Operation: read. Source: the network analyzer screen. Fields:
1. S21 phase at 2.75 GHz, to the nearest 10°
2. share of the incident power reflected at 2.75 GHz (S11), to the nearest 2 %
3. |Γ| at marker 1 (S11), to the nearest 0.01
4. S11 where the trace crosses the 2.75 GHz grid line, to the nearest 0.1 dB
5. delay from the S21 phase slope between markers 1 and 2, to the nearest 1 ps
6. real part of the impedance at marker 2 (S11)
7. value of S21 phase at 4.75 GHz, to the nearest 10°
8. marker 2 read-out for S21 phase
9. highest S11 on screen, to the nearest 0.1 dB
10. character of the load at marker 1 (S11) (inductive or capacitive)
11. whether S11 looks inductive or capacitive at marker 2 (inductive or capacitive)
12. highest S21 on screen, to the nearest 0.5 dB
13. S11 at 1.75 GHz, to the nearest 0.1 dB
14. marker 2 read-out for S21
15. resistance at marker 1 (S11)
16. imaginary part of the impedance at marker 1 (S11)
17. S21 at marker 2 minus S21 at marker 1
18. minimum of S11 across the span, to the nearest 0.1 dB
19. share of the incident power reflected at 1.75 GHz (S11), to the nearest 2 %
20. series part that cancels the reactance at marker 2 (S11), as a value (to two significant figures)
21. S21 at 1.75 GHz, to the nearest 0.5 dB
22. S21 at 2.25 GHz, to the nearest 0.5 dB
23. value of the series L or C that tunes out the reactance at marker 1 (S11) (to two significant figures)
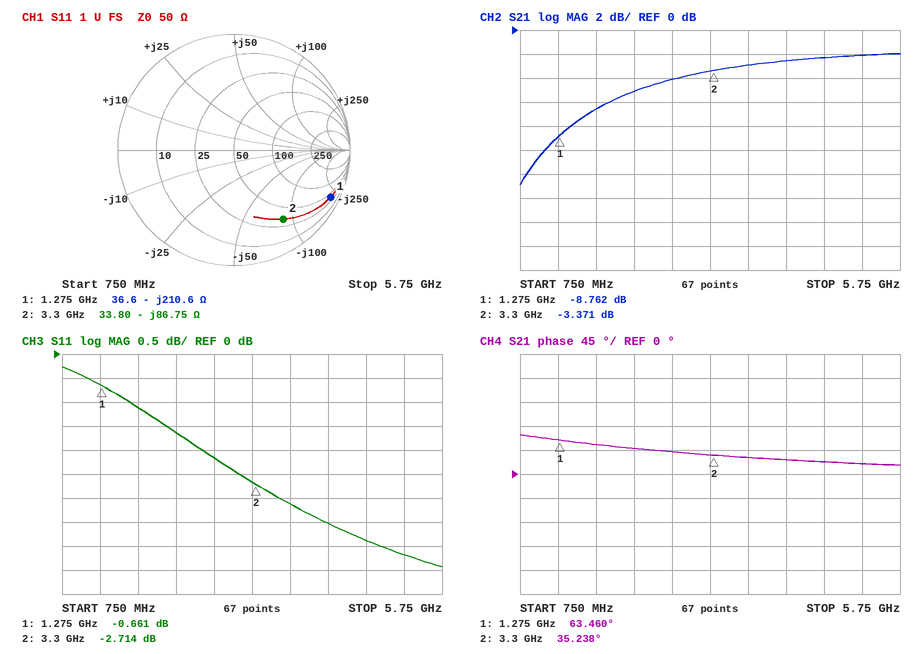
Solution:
40°
60 %
0.93
-2.2 dB
39 ps
33.80 Ω
20°
35.238°
-0.3 dB
capacitive
capacitive
-2.0 dB
-1.1 dB
-3.371 dB
36.6 Ω
-210.6 Ω
5.391 dB
-4.4 dB
78 %
4.2 nH
-6.5 dB
-5.0 dB
26 nH
